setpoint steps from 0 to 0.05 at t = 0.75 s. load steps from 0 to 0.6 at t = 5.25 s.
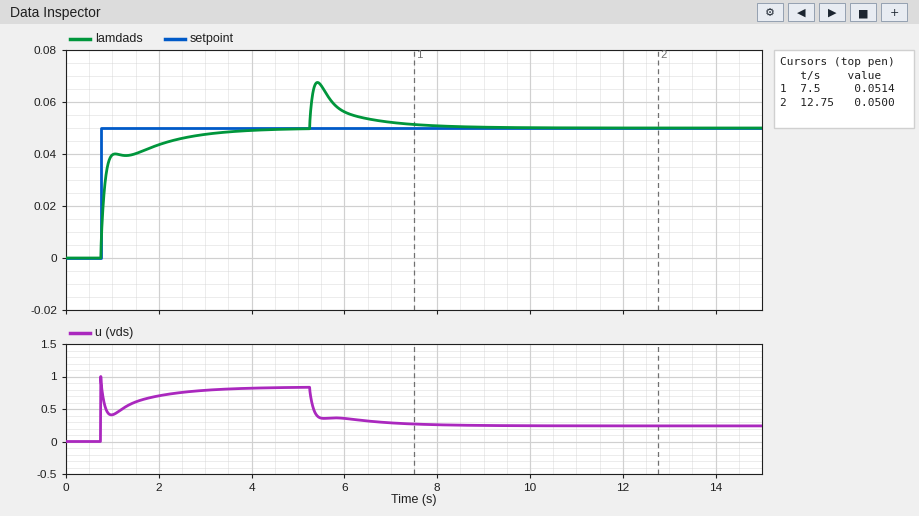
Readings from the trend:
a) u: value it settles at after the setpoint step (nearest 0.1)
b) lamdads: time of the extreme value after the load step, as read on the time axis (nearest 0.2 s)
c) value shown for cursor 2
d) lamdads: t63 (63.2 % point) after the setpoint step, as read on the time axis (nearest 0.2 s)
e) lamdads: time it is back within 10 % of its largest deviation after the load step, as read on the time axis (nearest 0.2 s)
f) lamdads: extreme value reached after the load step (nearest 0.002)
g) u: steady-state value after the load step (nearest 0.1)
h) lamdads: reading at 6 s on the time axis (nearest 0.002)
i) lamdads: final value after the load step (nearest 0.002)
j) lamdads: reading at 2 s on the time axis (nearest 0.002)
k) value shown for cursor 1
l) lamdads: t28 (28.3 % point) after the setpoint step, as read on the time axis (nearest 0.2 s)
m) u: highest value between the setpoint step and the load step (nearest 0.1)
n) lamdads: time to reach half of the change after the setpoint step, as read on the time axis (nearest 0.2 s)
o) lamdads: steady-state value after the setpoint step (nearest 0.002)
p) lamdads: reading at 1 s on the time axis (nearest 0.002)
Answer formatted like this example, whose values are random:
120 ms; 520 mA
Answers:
0.8; 5.4 s; 0.0500; 0.8 s; 7.2 s; 0.068; 0.2; 0.056; 0.050; 0.044; 0.0514; 0.8 s; 1.0; 0.8 s; 0.050; 0.040
